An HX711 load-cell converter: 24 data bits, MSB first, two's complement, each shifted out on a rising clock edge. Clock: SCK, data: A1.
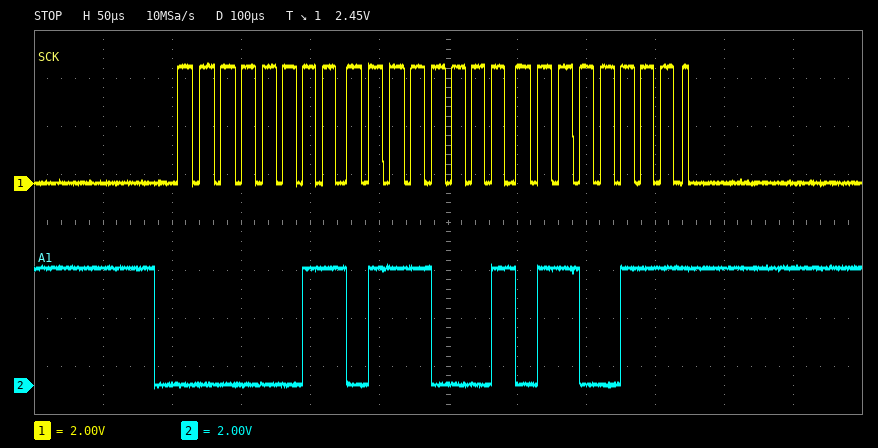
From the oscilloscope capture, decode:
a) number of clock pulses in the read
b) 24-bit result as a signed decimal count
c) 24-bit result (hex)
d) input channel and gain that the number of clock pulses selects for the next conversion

25
225639
0x037167
channel A, gain 128
